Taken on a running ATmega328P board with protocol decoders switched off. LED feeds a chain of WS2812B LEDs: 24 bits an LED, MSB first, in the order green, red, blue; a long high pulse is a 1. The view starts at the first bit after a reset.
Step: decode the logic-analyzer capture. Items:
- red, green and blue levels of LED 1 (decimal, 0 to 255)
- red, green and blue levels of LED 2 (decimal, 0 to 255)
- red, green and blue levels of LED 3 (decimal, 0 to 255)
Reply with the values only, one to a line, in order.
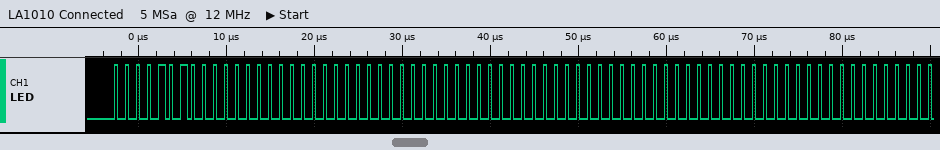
0, 10, 0
0, 0, 0
0, 0, 0
